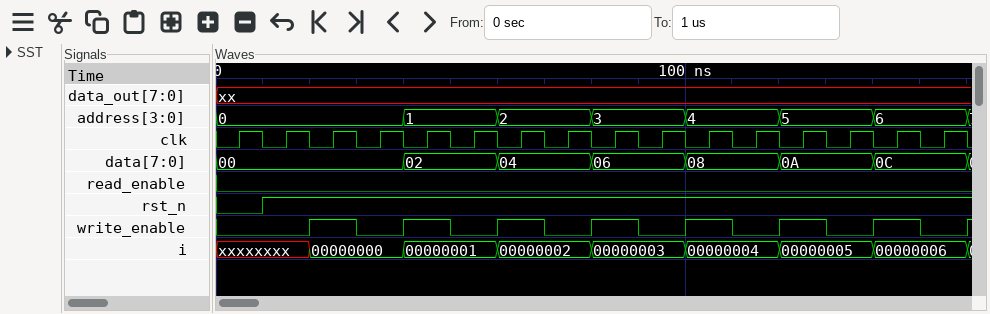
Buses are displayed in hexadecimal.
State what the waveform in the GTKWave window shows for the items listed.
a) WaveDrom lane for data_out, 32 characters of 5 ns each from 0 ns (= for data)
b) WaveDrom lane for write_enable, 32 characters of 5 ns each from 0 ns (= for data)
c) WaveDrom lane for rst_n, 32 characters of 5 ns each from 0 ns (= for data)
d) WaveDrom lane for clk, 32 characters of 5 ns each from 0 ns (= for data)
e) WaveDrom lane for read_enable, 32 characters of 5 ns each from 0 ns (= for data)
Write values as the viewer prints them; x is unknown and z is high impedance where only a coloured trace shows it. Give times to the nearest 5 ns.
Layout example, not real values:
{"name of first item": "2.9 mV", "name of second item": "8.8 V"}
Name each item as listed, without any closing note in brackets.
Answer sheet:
{"WaveDrom lane for data_out, 32 characters of 5 ns each from 0 ns": "{name: 'data_out', wave: 'x...............................'}", "WaveDrom lane for write_enable, 32 characters of 5 ns each from 0 ns": "{name: 'write_enable', wave: '0...1.0.1.0.1.0.1.0.1.0.1.0.1.0.'}", "WaveDrom lane for rst_n, 32 characters of 5 ns each from 0 ns": "{name: 'rst_n', wave: '0.1.............................'}", "WaveDrom lane for clk, 32 characters of 5 ns each from 0 ns": "{name: 'clk', wave: '01010101010101010101010101010101'}", "WaveDrom lane for read_enable, 32 characters of 5 ns each from 0 ns": "{name: 'read_enable', wave: '0...............................'}"}
